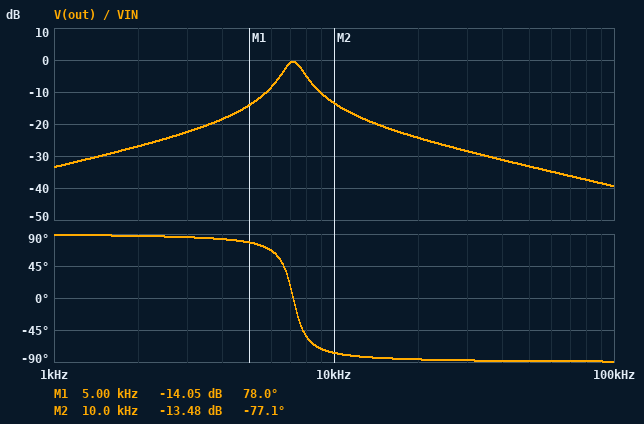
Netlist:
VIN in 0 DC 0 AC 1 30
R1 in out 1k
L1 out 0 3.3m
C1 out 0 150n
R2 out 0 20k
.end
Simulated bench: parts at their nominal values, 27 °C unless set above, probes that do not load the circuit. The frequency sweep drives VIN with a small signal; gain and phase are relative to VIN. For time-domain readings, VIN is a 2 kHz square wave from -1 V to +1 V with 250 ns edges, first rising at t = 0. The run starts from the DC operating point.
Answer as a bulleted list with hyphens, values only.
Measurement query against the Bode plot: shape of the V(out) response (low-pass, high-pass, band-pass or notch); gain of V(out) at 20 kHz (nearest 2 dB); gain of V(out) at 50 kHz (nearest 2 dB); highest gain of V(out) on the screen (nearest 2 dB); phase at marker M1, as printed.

- band-pass
- -24 dB
- -34 dB
- 0 dB
- 78.0 deg
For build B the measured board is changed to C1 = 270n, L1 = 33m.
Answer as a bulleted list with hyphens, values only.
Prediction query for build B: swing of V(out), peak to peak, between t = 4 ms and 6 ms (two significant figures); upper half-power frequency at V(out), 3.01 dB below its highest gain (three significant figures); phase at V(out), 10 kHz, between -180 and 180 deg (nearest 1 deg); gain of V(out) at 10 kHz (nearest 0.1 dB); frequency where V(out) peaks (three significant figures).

- 1.7 V
- 2.02 kHz
- -86 deg
- -24.4 dB
- 1.69 kHz
